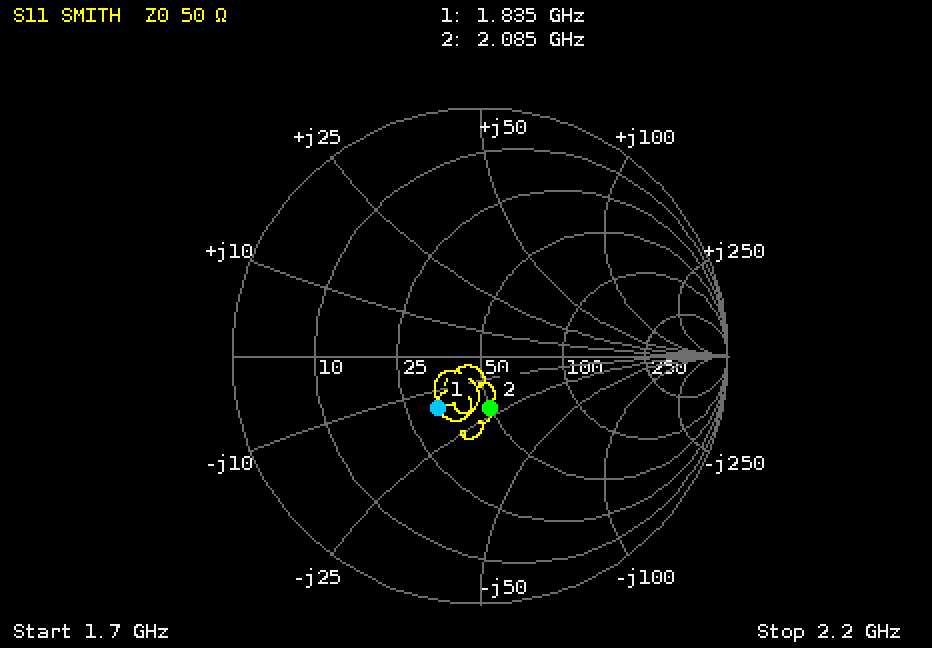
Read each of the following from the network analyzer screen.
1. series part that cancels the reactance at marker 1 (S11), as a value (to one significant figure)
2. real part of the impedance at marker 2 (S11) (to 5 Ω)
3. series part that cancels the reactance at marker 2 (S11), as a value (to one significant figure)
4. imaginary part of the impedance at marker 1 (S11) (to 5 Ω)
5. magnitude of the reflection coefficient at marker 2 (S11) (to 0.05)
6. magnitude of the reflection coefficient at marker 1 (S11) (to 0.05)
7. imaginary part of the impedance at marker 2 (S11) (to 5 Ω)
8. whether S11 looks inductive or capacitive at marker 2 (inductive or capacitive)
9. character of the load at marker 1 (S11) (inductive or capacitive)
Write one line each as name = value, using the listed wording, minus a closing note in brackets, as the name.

series part that cancels the reactance at marker 1 (S11), as a value = 1 nH
real part of the impedance at marker 2 (S11) = 50 Ω
series part that cancels the reactance at marker 2 (S11), as a value = 2 nH
imaginary part of the impedance at marker 1 (S11) = -15 Ω
magnitude of the reflection coefficient at marker 2 (S11) = 0.20
magnitude of the reflection coefficient at marker 1 (S11) = 0.25
imaginary part of the impedance at marker 2 (S11) = -20 Ω
whether S11 looks inductive or capacitive at marker 2 = capacitive
character of the load at marker 1 (S11) = capacitive
